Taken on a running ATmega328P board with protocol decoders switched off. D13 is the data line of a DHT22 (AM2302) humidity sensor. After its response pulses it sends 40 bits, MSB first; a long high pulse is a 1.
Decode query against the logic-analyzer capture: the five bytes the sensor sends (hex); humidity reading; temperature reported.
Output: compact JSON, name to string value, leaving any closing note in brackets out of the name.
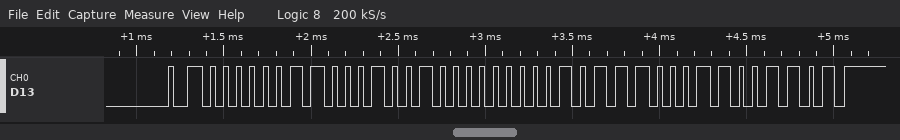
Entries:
{"the five bytes the sensor sends": "03 12 00 B8 CD", "humidity reading": "78.6 %", "temperature reported": "18.4 °C"}
